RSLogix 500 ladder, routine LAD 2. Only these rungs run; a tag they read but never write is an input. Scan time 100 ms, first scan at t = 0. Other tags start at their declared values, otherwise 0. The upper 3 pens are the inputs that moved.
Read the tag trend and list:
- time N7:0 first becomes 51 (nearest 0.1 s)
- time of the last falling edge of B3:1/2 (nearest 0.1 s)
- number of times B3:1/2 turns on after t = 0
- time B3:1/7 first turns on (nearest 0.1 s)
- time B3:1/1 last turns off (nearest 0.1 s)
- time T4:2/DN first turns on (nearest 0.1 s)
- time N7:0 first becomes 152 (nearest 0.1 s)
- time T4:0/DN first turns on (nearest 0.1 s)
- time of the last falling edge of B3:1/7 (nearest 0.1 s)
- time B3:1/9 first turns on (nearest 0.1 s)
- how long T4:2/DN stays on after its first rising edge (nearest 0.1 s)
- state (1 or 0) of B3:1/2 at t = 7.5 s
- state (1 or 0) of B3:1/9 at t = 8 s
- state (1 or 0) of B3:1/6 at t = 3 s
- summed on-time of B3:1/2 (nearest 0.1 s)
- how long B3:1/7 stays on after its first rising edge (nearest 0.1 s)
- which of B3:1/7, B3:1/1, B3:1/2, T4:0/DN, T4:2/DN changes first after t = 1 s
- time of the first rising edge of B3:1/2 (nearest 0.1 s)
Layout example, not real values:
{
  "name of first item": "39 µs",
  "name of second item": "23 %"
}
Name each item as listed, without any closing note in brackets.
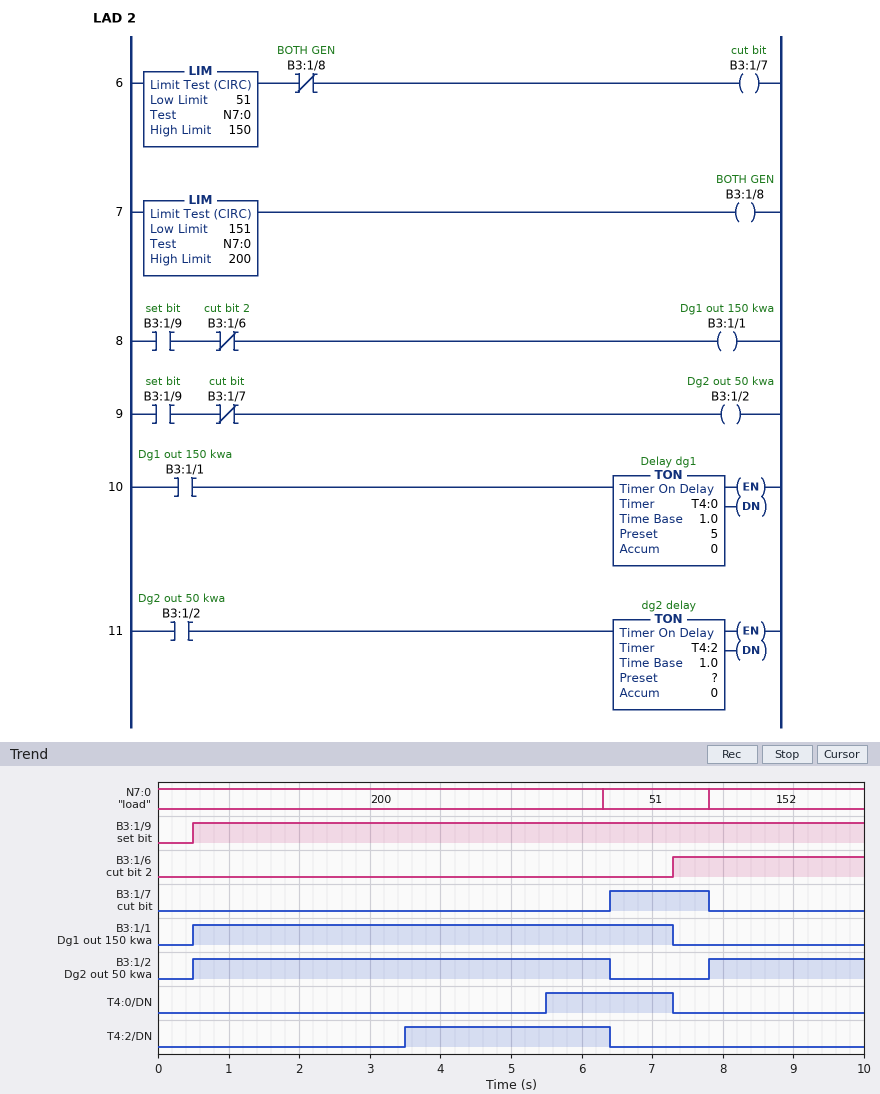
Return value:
{
  "time N7:0 first becomes 51": "6.3 s",
  "time of the last falling edge of B3:1/2": "6.4 s",
  "number of times B3:1/2 turns on after t = 0": "2",
  "time B3:1/7 first turns on": "6.4 s",
  "time B3:1/1 last turns off": "7.3 s",
  "time T4:2/DN first turns on": "3.5 s",
  "time N7:0 first becomes 152": "7.8 s",
  "time T4:0/DN first turns on": "5.5 s",
  "time of the last falling edge of B3:1/7": "7.8 s",
  "time B3:1/9 first turns on": "0.5 s",
  "how long T4:2/DN stays on after its first rising edge": "2.9 s",
  "state (1 or 0) of B3:1/2 at t = 7.5 s": "0",
  "state (1 or 0) of B3:1/9 at t = 8 s": "1",
  "state (1 or 0) of B3:1/6 at t = 3 s": "0",
  "summed on-time of B3:1/2": "8.1 s",
  "how long B3:1/7 stays on after its first rising edge": "1.4 s",
  "which of B3:1/7, B3:1/1, B3:1/2, T4:0/DN, T4:2/DN changes first after t = 1 s": "T4:2/DN",
  "time of the first rising edge of B3:1/2": "0.5 s"
}
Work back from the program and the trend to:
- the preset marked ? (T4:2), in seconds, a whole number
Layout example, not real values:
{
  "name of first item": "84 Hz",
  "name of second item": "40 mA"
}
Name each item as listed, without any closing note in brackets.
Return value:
{
  "the preset marked ? (T4:2), in seconds, a whole number": "3 s"
}
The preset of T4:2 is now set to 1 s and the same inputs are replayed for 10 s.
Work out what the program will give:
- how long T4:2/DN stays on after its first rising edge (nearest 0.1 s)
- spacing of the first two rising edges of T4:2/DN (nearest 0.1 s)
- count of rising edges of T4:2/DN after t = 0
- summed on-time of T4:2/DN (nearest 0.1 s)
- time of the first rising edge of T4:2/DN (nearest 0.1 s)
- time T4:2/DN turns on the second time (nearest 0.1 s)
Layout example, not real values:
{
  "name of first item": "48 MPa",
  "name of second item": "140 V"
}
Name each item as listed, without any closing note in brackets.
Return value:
{
  "how long T4:2/DN stays on after its first rising edge": "4.9 s",
  "spacing of the first two rising edges of T4:2/DN": "7.3 s",
  "count of rising edges of T4:2/DN after t = 0": "2",
  "summed on-time of T4:2/DN": "6.1 s",
  "time of the first rising edge of T4:2/DN": "1.5 s",
  "time T4:2/DN turns on the second time": "8.8 s"
}
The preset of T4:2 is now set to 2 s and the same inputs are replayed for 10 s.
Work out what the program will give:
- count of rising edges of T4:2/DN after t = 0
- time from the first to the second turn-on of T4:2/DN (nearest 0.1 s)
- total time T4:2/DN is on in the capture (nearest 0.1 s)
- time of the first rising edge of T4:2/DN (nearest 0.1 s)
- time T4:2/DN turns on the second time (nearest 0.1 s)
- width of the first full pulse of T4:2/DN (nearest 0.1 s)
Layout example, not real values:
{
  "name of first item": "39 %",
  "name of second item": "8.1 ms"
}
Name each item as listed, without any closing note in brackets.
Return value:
{
  "count of rising edges of T4:2/DN after t = 0": "2",
  "time from the first to the second turn-on of T4:2/DN": "7.3 s",
  "total time T4:2/DN is on in the capture": "4.1 s",
  "time of the first rising edge of T4:2/DN": "2.5 s",
  "time T4:2/DN turns on the second time": "9.8 s",
  "width of the first full pulse of T4:2/DN": "3.9 s"
}
